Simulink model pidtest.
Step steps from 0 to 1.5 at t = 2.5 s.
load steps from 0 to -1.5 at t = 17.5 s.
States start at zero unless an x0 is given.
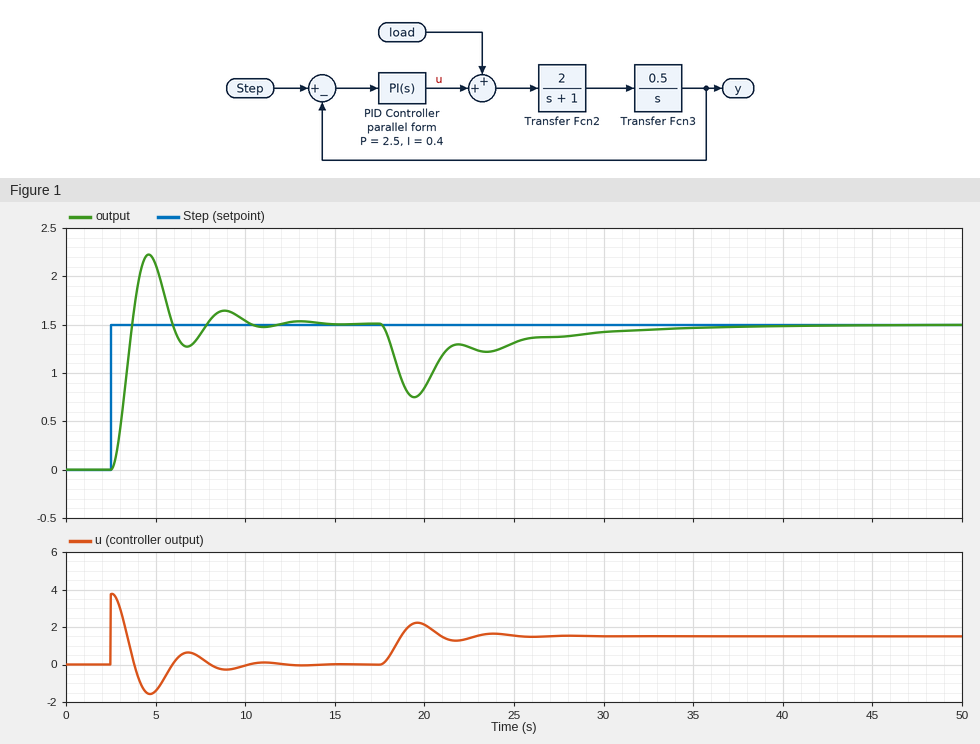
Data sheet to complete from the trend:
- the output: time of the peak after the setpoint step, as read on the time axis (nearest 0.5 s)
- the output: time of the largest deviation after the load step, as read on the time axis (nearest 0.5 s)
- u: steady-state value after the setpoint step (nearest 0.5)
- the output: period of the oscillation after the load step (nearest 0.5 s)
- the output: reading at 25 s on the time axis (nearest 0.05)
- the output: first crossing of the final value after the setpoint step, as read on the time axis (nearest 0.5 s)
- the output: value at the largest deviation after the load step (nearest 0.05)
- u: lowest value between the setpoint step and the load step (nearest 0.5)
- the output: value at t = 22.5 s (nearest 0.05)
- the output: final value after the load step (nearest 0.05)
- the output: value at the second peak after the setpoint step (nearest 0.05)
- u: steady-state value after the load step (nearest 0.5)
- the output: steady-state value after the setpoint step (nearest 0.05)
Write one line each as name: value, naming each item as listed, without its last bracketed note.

the output: time of the peak after the setpoint step, as read on the time axis: 4.5 s
the output: time of the largest deviation after the load step, as read on the time axis: 19.5 s
u: steady-state value after the setpoint step: 0.0
the output: period of the oscillation after the load step: 4.0 s
the output: reading at 25 s on the time axis: 1.30
the output: first crossing of the final value after the setpoint step, as read on the time axis: 3.5 s
the output: value at the largest deviation after the load step: 0.75
u: lowest value between the setpoint step and the load step: -1.5
the output: value at t = 22.5 s: 1.25
the output: final value after the load step: 1.50
the output: value at the second peak after the setpoint step: 1.65
u: steady-state value after the load step: 1.5
the output: steady-state value after the setpoint step: 1.50
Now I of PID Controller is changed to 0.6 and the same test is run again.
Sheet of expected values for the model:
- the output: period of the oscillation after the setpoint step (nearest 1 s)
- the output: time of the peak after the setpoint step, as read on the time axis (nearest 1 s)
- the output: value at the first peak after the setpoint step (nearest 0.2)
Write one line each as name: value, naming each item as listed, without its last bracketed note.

the output: period of the oscillation after the setpoint step: 4 s
the output: time of the peak after the setpoint step, as read on the time axis: 5 s
the output: value at the first peak after the setpoint step: 2.4
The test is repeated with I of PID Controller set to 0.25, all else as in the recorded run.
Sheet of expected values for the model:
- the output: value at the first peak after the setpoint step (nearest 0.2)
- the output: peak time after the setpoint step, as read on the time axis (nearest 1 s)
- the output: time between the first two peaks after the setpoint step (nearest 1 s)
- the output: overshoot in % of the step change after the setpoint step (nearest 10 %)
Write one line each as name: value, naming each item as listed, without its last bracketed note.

the output: value at the first peak after the setpoint step: 2.2
the output: peak time after the setpoint step, as read on the time axis: 5 s
the output: time between the first two peaks after the setpoint step: 4 s
the output: overshoot in % of the step change after the setpoint step: 40 %
